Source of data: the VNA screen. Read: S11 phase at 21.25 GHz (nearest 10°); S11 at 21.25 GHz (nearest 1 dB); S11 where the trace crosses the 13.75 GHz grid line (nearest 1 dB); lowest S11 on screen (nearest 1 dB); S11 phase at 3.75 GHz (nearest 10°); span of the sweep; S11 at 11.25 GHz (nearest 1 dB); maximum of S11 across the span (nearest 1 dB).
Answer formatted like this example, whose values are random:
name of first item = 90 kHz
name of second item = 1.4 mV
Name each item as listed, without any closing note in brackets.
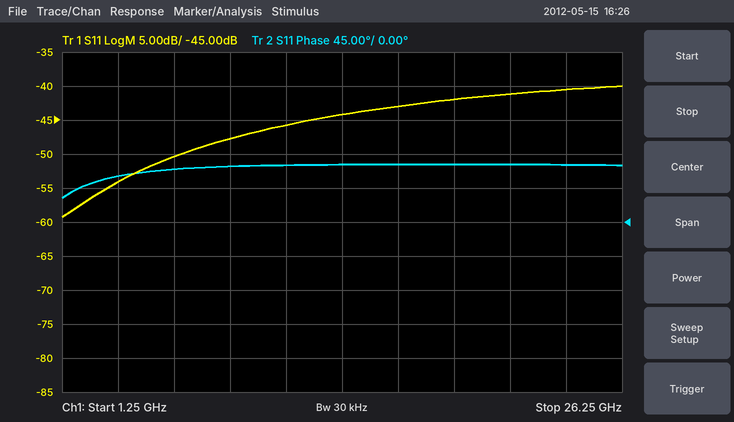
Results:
S11 phase at 21.25 GHz = 80°
S11 at 21.25 GHz = -41 dB
S11 where the trace crosses the 13.75 GHz grid line = -44 dB
lowest S11 on screen = -59 dB
S11 phase at 3.75 GHz = 60°
span of the sweep = 25 GHz
S11 at 11.25 GHz = -46 dB
maximum of S11 across the span = -40 dB
